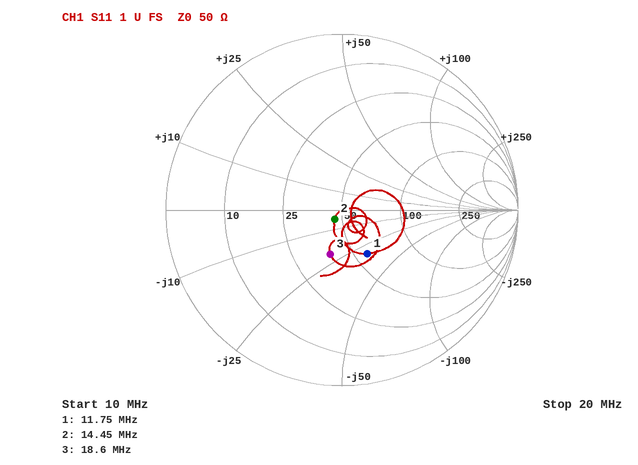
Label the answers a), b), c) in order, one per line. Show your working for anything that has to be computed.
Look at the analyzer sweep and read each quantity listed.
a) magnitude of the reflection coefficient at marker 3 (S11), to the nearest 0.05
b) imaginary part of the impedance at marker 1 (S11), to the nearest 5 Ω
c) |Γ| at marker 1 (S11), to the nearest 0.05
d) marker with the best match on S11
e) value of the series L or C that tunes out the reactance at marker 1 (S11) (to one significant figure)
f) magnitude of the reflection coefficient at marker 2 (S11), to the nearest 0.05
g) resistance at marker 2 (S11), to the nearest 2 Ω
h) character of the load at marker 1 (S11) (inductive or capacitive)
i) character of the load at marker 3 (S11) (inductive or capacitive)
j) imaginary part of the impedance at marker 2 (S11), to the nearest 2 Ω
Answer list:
a) 0.25
b) -30 Ω
c) 0.30
d) marker 2
e) L = 30 Ω/(2π × 11.75 MHz) ≈ 406 nH, so 400 nH to one significant figure
f) 0.05
g) 46 Ω
h) capacitive
i) capacitive
j) -4 Ω
